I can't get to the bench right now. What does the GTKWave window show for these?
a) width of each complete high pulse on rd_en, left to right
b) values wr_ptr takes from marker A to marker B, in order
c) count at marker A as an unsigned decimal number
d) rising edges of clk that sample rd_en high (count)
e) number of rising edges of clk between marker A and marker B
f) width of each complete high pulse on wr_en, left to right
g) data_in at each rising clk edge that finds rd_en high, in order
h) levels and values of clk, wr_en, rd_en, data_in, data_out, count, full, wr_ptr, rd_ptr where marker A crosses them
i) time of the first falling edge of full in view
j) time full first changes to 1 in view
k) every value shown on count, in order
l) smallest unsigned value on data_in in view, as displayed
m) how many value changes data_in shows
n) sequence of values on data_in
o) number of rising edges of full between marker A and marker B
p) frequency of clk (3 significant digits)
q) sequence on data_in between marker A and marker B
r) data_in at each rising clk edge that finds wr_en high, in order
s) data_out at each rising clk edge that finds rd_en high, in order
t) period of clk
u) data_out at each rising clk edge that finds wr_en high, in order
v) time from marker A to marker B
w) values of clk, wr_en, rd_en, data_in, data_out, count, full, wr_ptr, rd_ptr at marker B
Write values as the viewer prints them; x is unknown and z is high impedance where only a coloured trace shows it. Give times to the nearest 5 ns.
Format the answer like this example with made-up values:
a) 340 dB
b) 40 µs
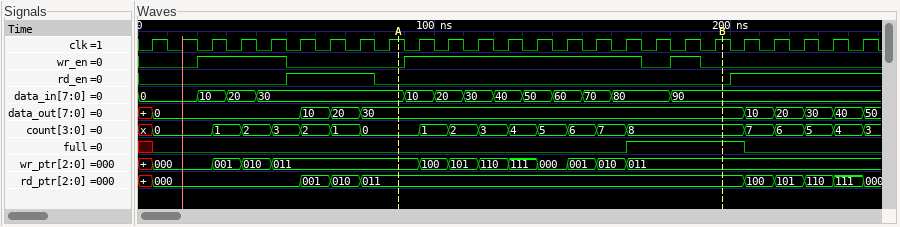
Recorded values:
a) 30 ns
b) 011, 100, 101, 110, 111, 000, 001, 010, 011
c) 0
d) 8
e) 11
f) 30 ns, 80 ns, 10 ns
g) 30, 30, 30, 90, 90, 90, 90, 90
h) clk=1, wr_en=0, rd_en=0, data_in=30, data_out=30, count=0, full=0, wr_ptr=011, rd_ptr=011
i) 205 ns
j) 165 ns
k) x, 0, 1, 2, 3, 2, 1, 0, 1, 2, 3, 4, 5, 6, 7, 8, 7, 6, 5, 4, 3
l) 0
m) 12
n) 0, 10, 20, 30, 10, 20, 30, 40, 50, 60, 70, 80, 90
o) 1
p) 100 MHz
q) 30, 10, 20, 30, 40, 50, 60, 70, 80, 90
r) 10, 20, 30, 10, 20, 30, 40, 50, 60, 70, 80, 90
s) 0, 10, 20, 30, 10, 20, 30, 40
t) 10 ns
u) 0, 0, 0, 30, 30, 30, 30, 30, 30, 30, 30, 30
v) 110 ns
w) clk=1, wr_en=0, rd_en=0, data_in=90, data_out=30, count=8, full=1, wr_ptr=011, rd_ptr=011
